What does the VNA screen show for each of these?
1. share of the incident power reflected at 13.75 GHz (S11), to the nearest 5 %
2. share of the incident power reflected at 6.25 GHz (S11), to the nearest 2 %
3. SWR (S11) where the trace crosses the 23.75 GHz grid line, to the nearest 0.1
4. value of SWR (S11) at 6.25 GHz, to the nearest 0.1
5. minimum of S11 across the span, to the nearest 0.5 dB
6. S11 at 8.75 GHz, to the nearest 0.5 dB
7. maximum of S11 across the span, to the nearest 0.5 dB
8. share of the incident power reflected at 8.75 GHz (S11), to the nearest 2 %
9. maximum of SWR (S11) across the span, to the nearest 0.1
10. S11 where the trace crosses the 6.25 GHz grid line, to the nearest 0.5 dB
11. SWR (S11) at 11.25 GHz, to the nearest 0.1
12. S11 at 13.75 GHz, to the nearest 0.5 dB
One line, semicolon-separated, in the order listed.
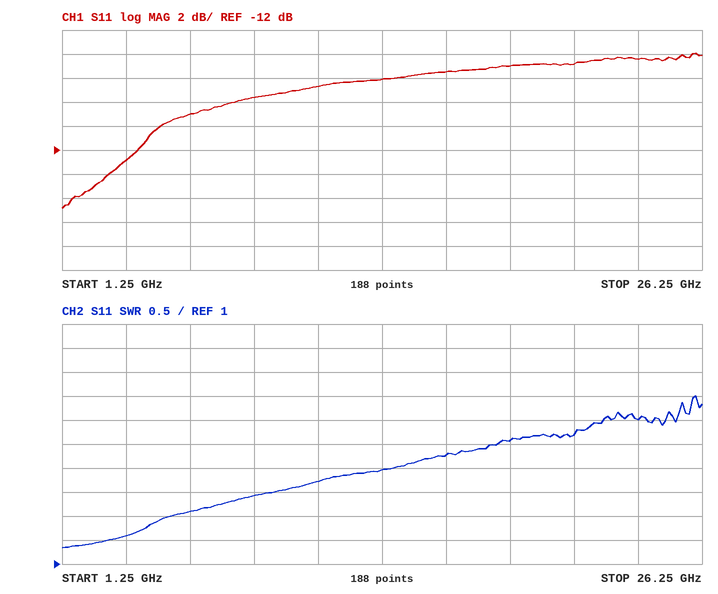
25 %; 12 %; 4.0; 2.1; -17.0 dB; -7.5 dB; -4.0 dB; 18 %; 4.5; -9.0 dB; 2.7; -6.0 dB
